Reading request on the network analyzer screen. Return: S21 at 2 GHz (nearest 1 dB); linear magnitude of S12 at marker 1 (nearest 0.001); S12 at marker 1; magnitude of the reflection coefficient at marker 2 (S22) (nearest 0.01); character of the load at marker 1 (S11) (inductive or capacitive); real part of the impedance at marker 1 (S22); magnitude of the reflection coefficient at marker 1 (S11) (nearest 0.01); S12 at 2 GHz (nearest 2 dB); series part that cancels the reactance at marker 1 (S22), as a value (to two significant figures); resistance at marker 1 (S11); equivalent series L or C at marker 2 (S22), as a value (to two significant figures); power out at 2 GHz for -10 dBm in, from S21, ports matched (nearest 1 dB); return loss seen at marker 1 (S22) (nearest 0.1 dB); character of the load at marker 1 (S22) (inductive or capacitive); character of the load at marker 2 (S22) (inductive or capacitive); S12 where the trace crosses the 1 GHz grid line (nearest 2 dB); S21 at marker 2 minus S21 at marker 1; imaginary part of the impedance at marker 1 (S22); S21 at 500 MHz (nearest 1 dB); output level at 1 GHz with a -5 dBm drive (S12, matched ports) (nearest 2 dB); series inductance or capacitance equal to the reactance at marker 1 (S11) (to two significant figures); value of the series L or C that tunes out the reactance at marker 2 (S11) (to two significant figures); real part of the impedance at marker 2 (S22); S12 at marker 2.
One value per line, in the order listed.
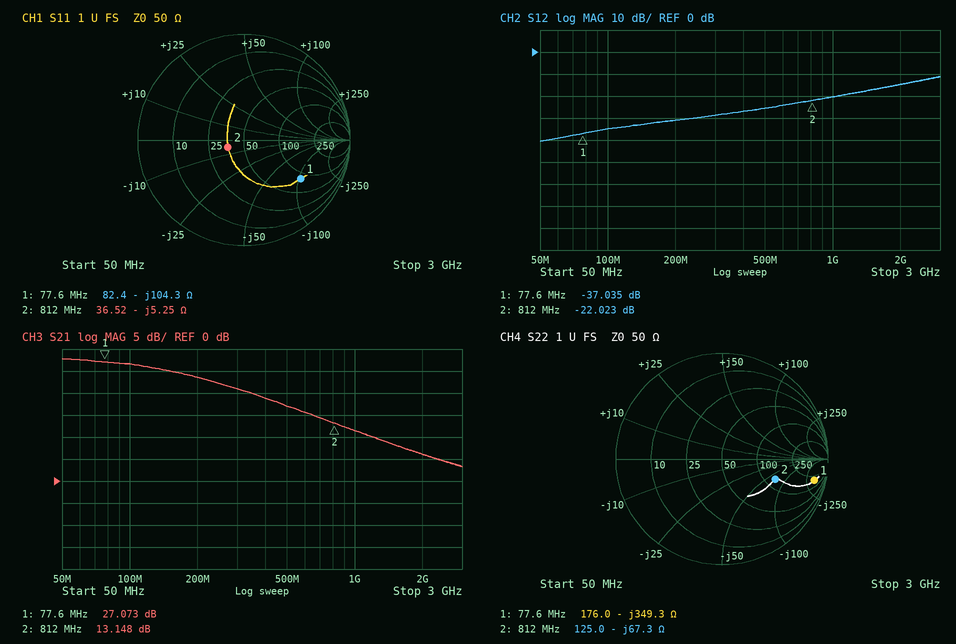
6 dB
0.014
-37.035 dB
0.54
capacitive
176.0 Ω
0.65
-14 dB
720 nH
82.4 Ω
2.9 pF
-4 dBm
1.0 dB
capacitive
capacitive
-20 dB
-13.925 dB
-349.3 Ω
17 dB
-26 dBm
20 pF
1.0 nH
125.0 Ω
-22.023 dB
